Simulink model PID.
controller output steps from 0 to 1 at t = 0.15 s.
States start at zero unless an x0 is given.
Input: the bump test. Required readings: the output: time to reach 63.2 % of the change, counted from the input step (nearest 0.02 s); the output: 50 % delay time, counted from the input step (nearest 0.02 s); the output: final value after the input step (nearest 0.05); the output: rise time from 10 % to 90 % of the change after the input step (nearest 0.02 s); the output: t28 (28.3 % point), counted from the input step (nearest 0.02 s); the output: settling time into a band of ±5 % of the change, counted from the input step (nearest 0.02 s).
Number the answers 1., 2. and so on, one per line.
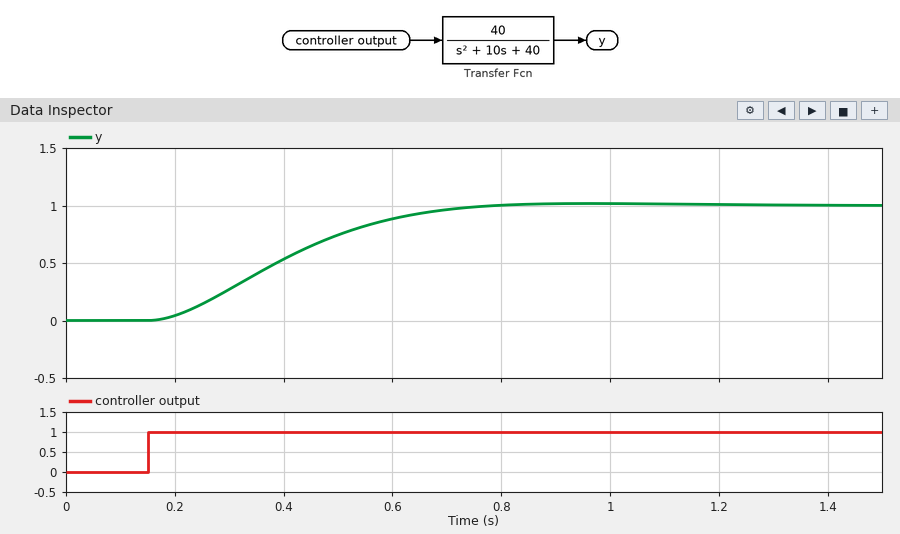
1. 0.30 s
2. 0.24 s
3. 1.00
4. 0.38 s
5. 0.16 s
6. 0.52 s
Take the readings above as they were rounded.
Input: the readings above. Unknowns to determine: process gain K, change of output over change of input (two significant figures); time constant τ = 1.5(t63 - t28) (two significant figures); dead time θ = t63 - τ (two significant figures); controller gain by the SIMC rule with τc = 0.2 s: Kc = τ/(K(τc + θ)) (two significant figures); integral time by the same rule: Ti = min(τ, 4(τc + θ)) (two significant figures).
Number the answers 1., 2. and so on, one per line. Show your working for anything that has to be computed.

1. (1 - 0) / 1 = 1.0
2. 1.5 × (0.3 - 0.16) = 0.21 s
3. 0.3 - 0.21 = 0.090 s
4. 0.21 / (1 × (0.2 + 0.09)) = 0.72
5. min(0.21, 4 × (0.2 + 0.09)) = 0.21 s
